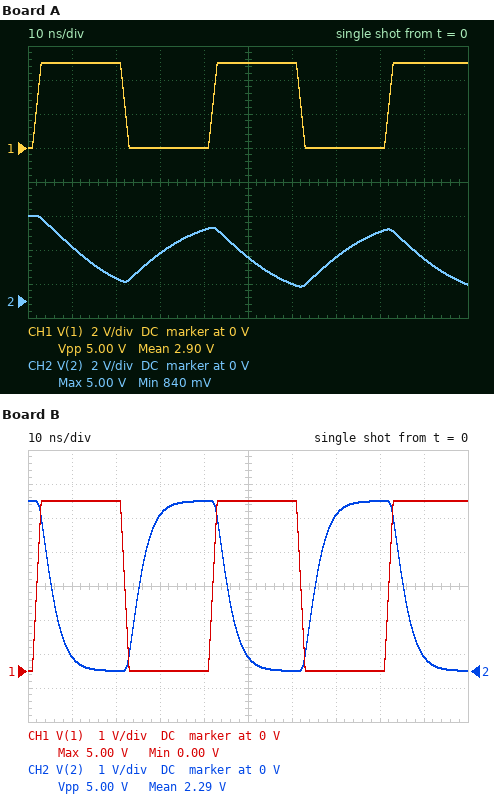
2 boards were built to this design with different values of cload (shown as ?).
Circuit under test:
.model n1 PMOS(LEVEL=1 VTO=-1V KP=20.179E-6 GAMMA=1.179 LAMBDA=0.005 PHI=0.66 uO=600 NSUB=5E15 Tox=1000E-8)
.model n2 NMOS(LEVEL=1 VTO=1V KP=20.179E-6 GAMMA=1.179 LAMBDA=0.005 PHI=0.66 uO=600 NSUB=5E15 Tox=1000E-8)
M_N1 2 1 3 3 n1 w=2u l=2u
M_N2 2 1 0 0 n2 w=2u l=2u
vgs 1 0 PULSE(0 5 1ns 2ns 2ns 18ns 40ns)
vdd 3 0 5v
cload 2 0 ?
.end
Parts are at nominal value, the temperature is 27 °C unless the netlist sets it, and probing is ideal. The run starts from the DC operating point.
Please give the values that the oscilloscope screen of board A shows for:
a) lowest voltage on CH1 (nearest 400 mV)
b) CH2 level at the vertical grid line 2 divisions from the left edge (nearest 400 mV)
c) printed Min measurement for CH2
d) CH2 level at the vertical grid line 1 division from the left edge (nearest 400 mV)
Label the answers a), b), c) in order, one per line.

a) 0 V
b) 1.2 V
c) 840 mV
d) 3.2 V
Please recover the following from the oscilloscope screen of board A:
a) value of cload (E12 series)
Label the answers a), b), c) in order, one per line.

a) 680 fF
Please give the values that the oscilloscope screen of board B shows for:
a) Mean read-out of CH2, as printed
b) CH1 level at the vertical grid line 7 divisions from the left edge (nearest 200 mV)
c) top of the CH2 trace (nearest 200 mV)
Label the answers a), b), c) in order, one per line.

a) 2.29 V
b) 0 V
c) 5.0 V
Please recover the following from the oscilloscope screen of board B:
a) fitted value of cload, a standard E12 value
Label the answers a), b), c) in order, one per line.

a) 180 fF
